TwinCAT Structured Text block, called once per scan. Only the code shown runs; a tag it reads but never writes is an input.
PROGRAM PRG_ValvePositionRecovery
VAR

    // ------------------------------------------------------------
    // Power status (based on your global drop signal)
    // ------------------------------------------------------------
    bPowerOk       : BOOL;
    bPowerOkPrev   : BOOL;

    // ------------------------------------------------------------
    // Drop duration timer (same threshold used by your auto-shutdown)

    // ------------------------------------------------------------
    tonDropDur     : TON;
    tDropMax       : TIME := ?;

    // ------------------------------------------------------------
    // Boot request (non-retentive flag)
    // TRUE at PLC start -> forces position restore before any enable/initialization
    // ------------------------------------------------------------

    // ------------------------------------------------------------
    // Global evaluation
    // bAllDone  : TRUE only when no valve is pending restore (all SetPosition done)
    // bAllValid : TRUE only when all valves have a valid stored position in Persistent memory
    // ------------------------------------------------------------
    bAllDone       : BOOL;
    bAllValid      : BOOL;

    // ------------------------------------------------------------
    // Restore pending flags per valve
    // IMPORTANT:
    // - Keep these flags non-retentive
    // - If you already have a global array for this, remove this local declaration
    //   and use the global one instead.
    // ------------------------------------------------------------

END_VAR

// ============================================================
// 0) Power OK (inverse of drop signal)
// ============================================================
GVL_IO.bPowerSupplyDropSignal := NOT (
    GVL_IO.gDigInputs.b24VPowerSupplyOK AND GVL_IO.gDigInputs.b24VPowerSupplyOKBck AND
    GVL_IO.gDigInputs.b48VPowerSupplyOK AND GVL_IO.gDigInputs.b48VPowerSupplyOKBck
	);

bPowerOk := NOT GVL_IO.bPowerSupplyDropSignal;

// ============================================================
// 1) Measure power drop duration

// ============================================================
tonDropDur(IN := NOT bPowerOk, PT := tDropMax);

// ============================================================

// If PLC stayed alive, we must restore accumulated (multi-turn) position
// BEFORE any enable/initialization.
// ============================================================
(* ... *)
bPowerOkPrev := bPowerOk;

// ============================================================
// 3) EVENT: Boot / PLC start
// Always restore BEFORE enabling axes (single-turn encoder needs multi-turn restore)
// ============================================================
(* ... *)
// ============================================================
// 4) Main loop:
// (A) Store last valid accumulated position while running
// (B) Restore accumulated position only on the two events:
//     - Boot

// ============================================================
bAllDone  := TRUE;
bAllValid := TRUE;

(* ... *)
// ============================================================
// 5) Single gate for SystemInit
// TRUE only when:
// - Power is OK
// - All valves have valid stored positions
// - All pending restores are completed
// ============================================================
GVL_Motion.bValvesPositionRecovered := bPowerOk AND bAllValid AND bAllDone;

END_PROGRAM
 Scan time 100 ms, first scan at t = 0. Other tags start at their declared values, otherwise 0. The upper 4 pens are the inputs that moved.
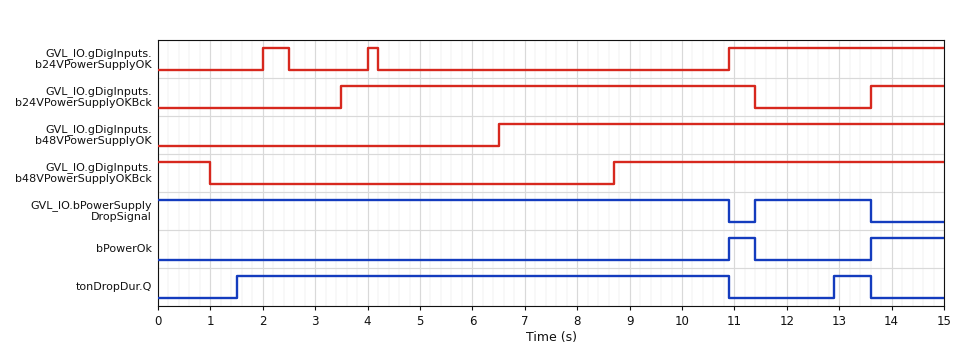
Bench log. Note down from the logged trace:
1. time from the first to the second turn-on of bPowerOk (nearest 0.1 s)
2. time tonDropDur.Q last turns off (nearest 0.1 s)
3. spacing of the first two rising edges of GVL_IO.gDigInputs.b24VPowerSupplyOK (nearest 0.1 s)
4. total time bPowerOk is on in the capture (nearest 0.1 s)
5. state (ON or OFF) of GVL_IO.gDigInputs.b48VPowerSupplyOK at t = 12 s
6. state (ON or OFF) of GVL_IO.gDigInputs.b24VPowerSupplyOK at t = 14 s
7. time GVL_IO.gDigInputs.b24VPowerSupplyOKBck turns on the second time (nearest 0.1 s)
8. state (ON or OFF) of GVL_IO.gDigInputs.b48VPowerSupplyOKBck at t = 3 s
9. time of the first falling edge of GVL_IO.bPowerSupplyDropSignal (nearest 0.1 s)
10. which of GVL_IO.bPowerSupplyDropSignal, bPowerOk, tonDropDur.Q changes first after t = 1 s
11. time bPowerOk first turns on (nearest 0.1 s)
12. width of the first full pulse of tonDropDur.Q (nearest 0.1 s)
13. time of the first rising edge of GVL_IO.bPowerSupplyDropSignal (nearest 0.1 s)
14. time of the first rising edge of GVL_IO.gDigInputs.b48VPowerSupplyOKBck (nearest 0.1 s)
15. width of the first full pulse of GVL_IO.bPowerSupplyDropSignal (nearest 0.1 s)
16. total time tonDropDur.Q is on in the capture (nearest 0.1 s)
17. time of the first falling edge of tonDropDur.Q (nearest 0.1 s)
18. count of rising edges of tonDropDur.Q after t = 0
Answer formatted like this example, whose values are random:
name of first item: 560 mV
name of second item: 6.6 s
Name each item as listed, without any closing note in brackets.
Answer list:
time from the first to the second turn-on of bPowerOk: 2.7 s
time tonDropDur.Q last turns off: 13.6 s
spacing of the first two rising edges of GVL_IO.gDigInputs.b24VPowerSupplyOK: 2.0 s
total time bPowerOk is on in the capture: 1.9 s
state (ON or OFF) of GVL_IO.gDigInputs.b48VPowerSupplyOK at t = 12 s: ON
state (ON or OFF) of GVL_IO.gDigInputs.b24VPowerSupplyOK at t = 14 s: ON
time GVL_IO.gDigInputs.b24VPowerSupplyOKBck turns on the second time: 13.6 s
state (ON or OFF) of GVL_IO.gDigInputs.b48VPowerSupplyOKBck at t = 3 s: OFF
time of the first falling edge of GVL_IO.bPowerSupplyDropSignal: 10.9 s
which of GVL_IO.bPowerSupplyDropSignal, bPowerOk, tonDropDur.Q changes first after t = 1 s: tonDropDur.Q
time bPowerOk first turns on: 10.9 s
width of the first full pulse of tonDropDur.Q: 9.4 s
time of the first rising edge of GVL_IO.bPowerSupplyDropSignal: 11.4 s
time of the first rising edge of GVL_IO.gDigInputs.b48VPowerSupplyOKBck: 8.7 s
width of the first full pulse of GVL_IO.bPowerSupplyDropSignal: 2.2 s
total time tonDropDur.Q is on in the capture: 10.1 s
time of the first falling edge of tonDropDur.Q: 10.9 s
count of rising edges of tonDropDur.Q after t = 0: 2
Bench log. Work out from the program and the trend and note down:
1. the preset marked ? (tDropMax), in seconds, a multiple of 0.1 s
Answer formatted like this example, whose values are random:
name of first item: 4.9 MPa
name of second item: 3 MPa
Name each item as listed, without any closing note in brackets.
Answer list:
the preset marked ? (tDropMax), in seconds, a multiple of 0.1 s: 1.5 s
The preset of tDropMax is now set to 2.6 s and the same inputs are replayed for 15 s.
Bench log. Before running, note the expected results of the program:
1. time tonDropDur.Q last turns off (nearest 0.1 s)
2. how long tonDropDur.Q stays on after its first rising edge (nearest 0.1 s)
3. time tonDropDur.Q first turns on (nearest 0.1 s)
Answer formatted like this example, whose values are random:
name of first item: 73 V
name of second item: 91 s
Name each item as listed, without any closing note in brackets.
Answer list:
time tonDropDur.Q last turns off: 10.9 s
how long tonDropDur.Q stays on after its first rising edge: 8.3 s
time tonDropDur.Q first turns on: 2.6 s
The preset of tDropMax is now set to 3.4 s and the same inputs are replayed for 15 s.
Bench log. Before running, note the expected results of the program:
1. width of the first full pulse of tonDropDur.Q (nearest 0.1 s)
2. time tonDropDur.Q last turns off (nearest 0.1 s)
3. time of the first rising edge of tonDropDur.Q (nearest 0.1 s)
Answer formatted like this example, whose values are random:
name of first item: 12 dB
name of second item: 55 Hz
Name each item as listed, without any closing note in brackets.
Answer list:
width of the first full pulse of tonDropDur.Q: 7.5 s
time tonDropDur.Q last turns off: 10.9 s
time of the first rising edge of tonDropDur.Q: 3.4 s
